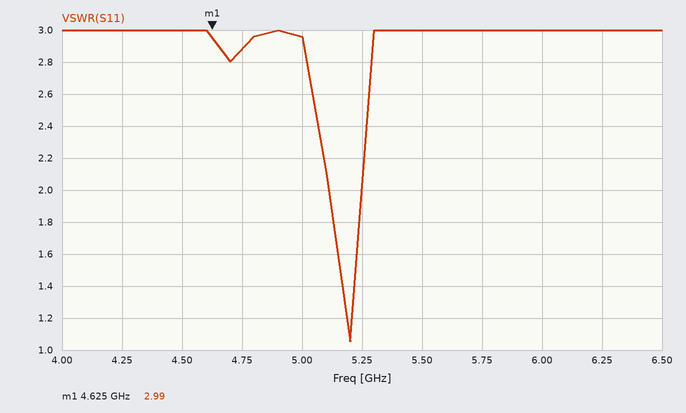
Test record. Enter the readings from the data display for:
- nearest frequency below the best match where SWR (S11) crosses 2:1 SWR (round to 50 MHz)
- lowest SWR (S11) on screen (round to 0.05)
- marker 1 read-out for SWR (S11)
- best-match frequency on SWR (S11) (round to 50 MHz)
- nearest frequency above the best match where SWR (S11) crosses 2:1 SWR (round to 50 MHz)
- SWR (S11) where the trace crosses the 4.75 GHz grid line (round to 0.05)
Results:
5.10 GHz
1.05
2.99
5.20 GHz
5.25 GHz
2.90
